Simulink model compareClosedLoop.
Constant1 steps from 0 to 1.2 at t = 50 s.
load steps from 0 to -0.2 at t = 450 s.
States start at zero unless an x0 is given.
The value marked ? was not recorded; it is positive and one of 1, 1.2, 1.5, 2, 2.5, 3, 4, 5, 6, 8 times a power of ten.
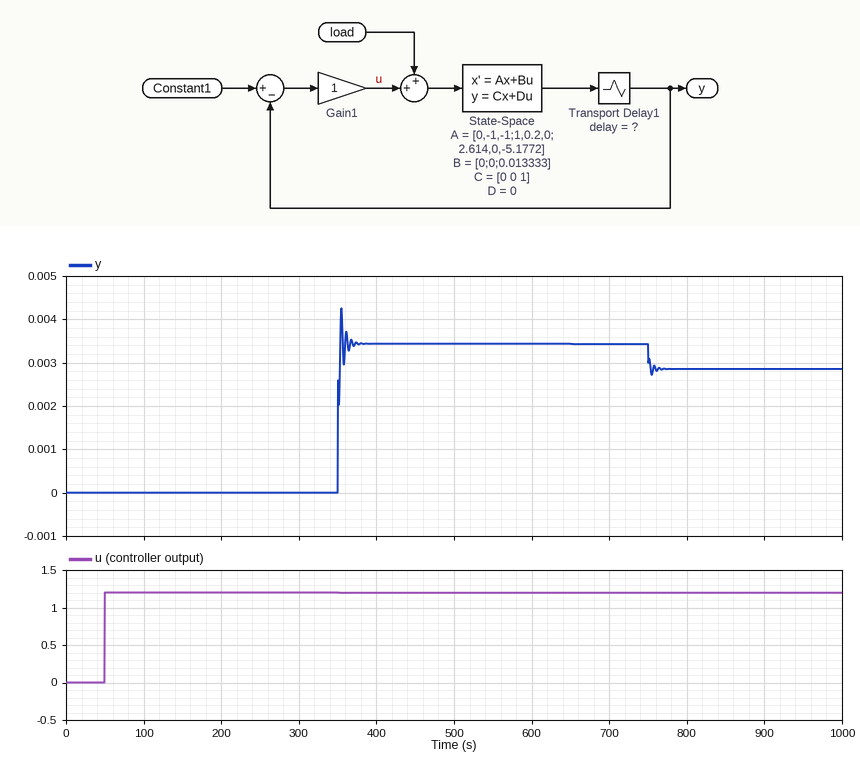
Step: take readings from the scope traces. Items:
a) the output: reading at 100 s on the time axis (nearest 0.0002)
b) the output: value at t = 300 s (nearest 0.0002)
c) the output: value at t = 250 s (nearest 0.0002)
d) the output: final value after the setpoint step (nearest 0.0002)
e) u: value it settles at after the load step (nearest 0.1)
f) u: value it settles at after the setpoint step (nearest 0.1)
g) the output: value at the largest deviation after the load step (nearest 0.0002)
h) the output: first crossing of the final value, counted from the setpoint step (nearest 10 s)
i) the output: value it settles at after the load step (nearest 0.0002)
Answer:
0.0000
0.0000
0.0000
0.0034
1.2
1.2
0.0028
300 s
0.0028
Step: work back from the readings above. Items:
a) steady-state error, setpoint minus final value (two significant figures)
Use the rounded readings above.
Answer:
1.2
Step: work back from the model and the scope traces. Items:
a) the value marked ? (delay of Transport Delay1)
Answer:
300
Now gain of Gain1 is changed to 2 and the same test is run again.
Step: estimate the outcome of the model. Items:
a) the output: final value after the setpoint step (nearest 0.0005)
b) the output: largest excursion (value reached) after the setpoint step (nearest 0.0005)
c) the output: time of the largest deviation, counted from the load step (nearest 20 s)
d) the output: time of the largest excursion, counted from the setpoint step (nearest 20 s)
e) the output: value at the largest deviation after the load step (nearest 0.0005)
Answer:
0.0070
0.0085
300 s
300 s
0.0060
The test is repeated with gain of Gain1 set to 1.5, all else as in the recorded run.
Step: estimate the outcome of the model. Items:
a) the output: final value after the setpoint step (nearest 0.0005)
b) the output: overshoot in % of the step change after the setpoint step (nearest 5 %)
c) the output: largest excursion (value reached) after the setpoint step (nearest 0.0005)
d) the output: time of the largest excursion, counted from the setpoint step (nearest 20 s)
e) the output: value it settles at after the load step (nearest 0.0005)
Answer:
0.0050
25 %
0.0065
300 s
0.0045
